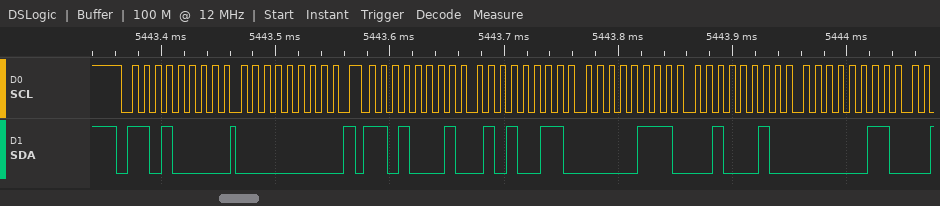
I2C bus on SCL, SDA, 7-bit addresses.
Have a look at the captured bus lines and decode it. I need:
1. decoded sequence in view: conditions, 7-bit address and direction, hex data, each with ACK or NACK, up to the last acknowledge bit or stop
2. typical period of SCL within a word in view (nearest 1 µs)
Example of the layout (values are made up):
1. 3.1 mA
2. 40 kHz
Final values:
1. start, address 68 write ACK, 00 ACK, repeated start, address 68 read ACK, 53 ACK, 07 ACK, 22 ACK, 03 ACK
2. 10 µs
